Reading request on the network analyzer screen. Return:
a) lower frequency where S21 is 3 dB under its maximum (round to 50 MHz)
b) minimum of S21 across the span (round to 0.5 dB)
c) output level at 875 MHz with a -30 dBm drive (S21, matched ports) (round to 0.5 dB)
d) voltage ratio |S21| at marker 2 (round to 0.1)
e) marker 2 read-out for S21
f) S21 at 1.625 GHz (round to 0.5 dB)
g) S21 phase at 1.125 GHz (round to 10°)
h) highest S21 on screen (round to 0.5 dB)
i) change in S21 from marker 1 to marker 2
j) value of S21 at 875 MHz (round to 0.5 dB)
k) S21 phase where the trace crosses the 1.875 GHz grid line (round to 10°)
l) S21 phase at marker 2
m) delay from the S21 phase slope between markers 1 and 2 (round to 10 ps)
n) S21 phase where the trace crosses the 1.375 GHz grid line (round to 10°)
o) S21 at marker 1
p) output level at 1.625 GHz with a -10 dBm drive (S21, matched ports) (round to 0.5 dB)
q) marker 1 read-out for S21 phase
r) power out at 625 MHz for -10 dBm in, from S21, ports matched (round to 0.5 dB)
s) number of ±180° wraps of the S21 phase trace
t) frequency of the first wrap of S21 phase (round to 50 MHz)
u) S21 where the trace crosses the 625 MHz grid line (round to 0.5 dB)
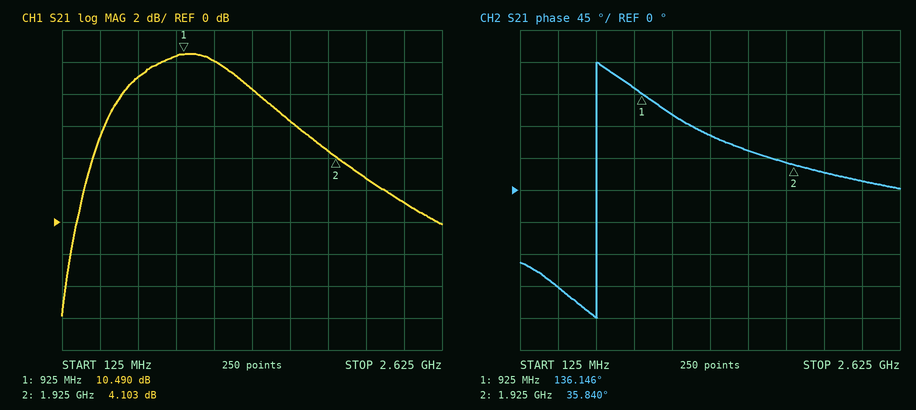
500 MHz
-6.0 dB
-19.5 dBm
1.6
4.103 dB
6.5 dB
110°
10.5 dB
-6.387 dB
10.5 dB
40°
35.840°
280 ps
80°
10.490 dB
-3.5 dBm
136.146°
-1.0 dBm
1
650 MHz
9.0 dB
